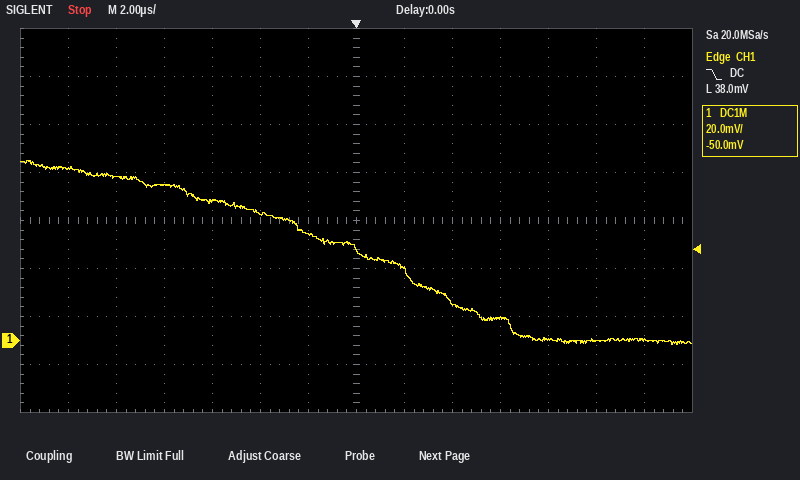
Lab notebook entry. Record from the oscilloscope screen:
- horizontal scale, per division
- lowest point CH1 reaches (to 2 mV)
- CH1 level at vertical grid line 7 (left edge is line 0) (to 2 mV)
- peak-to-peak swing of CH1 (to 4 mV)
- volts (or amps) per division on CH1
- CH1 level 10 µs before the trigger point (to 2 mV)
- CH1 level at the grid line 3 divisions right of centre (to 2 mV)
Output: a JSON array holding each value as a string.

["2 µs", "-2 mV", "38 mV", "76 mV", "20 mV", "68 mV", "10 mV"]
